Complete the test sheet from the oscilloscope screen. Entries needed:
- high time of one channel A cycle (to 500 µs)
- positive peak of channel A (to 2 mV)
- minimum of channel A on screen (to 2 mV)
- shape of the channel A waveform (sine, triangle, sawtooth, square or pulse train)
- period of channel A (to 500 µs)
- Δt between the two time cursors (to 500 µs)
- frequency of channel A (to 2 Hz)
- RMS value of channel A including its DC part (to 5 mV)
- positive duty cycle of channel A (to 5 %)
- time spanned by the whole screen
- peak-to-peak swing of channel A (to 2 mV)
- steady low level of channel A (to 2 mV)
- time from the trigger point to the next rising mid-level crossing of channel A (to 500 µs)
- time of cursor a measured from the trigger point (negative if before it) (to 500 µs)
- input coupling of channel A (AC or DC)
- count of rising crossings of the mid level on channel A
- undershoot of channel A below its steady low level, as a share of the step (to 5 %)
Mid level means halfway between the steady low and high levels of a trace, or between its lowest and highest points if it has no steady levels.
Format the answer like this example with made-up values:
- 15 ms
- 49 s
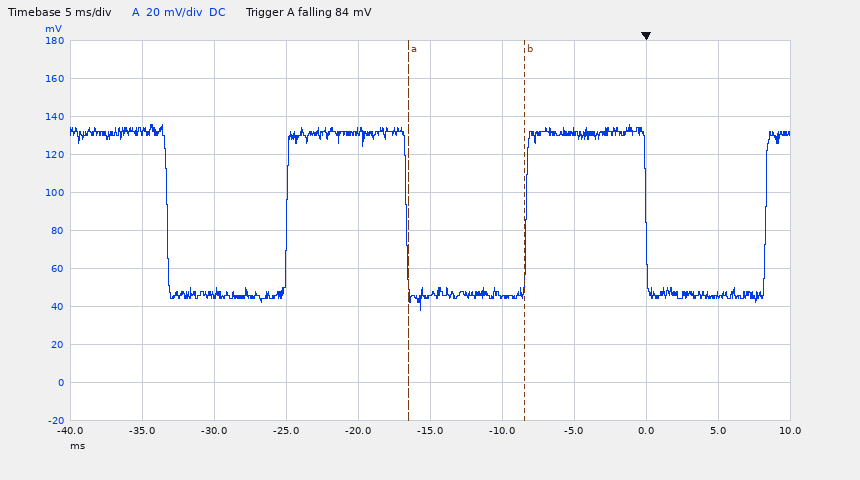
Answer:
- 8.5 ms
- 136 mV
- 38 mV
- square
- 16.5 ms
- 8.0 ms
- 60 Hz
- 100 mV
- 50 %
- 50 ms
- 98 mV
- 46 mV
- 8.5 ms
- -16.5 ms
- DC
- 3
- 10 %
